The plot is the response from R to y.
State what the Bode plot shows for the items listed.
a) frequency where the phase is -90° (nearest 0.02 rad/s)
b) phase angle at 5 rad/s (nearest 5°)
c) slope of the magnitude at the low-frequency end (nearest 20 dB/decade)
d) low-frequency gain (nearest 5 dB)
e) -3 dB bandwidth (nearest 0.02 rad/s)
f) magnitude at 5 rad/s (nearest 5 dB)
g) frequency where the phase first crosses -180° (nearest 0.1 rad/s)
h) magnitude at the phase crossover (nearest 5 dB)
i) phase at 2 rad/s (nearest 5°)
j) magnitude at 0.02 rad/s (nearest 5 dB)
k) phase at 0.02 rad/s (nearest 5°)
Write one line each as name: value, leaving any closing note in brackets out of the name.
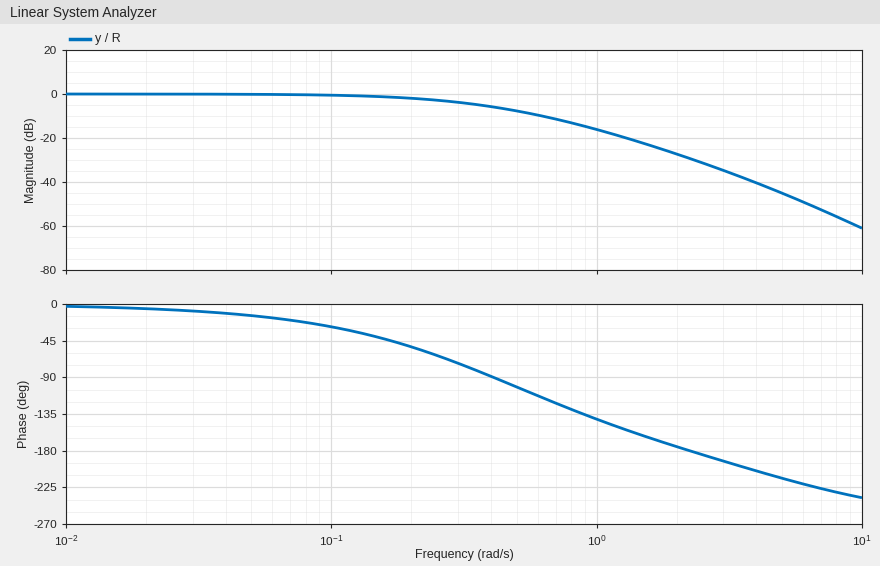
frequency where the phase is -90°: 0.40 rad/s
phase angle at 5 rad/s: -215°
slope of the magnitude at the low-frequency end: 0 dB/decade
low-frequency gain: 0 dB
-3 dB bandwidth: 0.26 rad/s
magnitude at 5 rad/s: -45 dB
frequency where the phase first crosses -180°: 2.2 rad/s
magnitude at the phase crossover: -30 dB
phase at 2 rad/s: -175°
magnitude at 0.02 rad/s: 0 dB
phase at 0.02 rad/s: -5°
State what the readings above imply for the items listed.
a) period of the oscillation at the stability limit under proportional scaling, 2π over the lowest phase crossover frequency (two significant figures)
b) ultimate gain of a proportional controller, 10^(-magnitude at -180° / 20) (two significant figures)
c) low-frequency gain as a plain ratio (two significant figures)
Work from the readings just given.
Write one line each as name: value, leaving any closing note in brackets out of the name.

period of the oscillation at the stability limit under proportional scaling, 2π over the lowest phase crossover frequency: 2.9 s
ultimate gain of a proportional controller, 10^(-magnitude at -180° / 20): 32
low-frequency gain as a plain ratio: 1.0
